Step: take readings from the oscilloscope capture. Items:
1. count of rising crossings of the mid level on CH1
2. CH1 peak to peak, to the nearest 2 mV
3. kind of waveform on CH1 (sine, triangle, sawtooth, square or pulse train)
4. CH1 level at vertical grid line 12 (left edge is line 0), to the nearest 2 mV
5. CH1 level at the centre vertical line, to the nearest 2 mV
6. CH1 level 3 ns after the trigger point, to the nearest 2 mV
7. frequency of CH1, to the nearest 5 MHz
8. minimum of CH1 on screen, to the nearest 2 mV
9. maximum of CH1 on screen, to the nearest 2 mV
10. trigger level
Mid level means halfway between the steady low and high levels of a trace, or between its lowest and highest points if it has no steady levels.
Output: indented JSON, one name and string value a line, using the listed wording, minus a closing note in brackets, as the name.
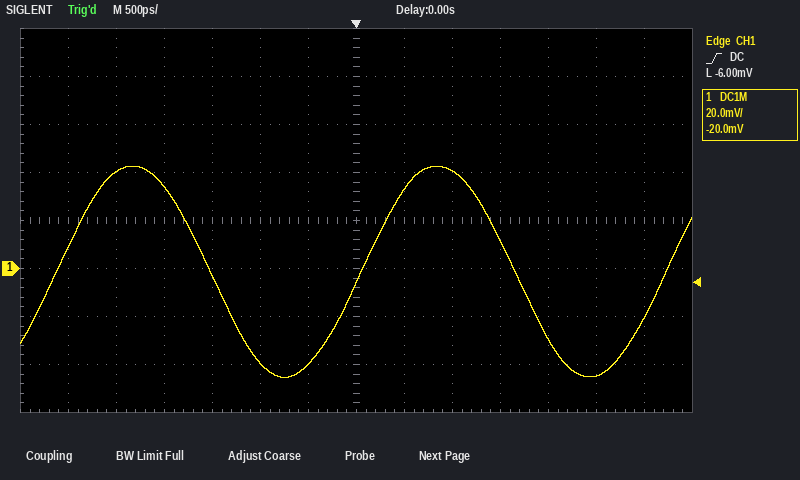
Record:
{
  "count of rising crossings of the mid level on CH1": "3",
  "CH1 peak to peak, to the nearest 2 mV": "88 mV",
  "kind of waveform on CH1": "sine",
  "CH1 level at vertical grid line 12 (left edge is line 0), to the nearest 2 mV": "-44 mV",
  "CH1 level at the centre vertical line, to the nearest 2 mV": "-6 mV",
  "CH1 level 3 ns after the trigger point, to the nearest 2 mV": "-20 mV",
  "frequency of CH1, to the nearest 5 MHz": "315 MHz",
  "minimum of CH1 on screen, to the nearest 2 mV": "-46 mV",
  "maximum of CH1 on screen, to the nearest 2 mV": "42 mV",
  "trigger level": "-6.00 mV"
}
